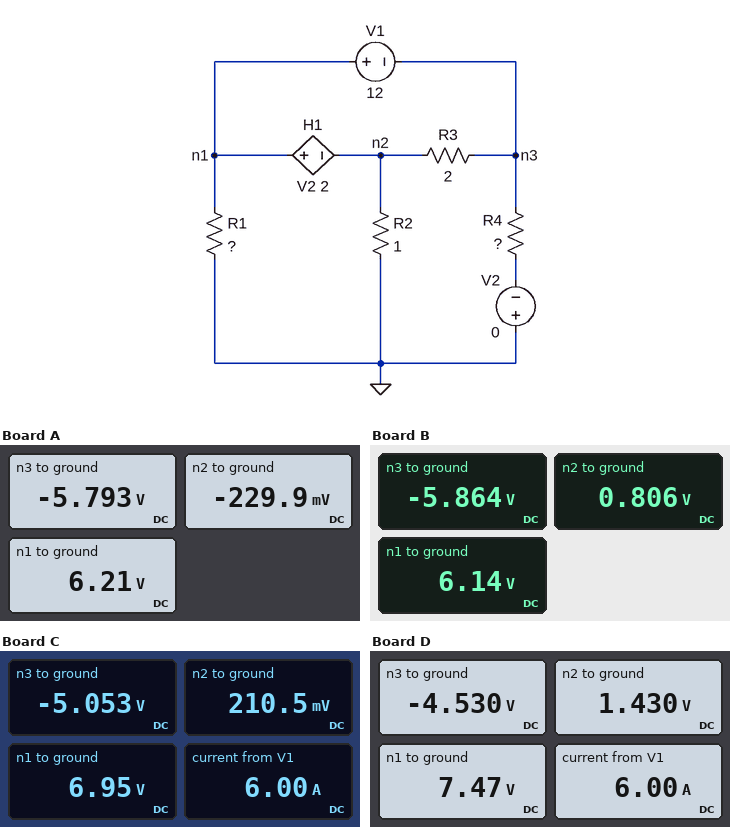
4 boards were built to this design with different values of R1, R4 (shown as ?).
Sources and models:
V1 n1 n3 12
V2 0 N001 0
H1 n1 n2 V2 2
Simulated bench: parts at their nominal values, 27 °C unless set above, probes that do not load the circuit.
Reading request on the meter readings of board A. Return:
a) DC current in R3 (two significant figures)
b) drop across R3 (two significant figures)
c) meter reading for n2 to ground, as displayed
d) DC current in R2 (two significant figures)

2.8 A
5.6 V
-229.9 mV
230 mA
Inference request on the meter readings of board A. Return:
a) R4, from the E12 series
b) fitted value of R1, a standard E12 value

1.8 Ω
1.8 Ω
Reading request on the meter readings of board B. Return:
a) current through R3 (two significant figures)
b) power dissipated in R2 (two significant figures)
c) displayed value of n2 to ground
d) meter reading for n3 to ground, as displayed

3.3 A
650 mW
0.806 V
-5.864 V
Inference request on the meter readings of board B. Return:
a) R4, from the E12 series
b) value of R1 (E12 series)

2.2 Ω
3.3 Ω
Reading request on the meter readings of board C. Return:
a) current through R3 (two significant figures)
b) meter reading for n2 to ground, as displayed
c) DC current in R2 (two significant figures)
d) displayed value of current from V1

2.6 A
210.5 mV
210 mA
6.00 A
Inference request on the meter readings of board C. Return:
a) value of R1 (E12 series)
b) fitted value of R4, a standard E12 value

2.2 Ω
1.5 Ω
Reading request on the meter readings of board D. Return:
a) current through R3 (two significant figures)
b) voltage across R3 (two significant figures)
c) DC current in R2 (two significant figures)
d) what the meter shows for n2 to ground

3.0 A
6.0 V
1.4 A
1.430 V
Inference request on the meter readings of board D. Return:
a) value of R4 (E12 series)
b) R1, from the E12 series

1.5 Ω
4.7 Ω
